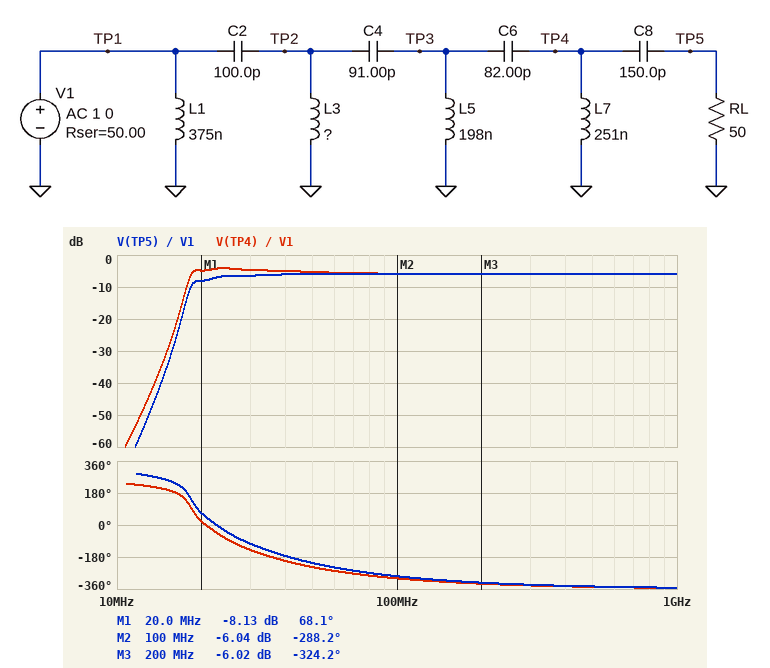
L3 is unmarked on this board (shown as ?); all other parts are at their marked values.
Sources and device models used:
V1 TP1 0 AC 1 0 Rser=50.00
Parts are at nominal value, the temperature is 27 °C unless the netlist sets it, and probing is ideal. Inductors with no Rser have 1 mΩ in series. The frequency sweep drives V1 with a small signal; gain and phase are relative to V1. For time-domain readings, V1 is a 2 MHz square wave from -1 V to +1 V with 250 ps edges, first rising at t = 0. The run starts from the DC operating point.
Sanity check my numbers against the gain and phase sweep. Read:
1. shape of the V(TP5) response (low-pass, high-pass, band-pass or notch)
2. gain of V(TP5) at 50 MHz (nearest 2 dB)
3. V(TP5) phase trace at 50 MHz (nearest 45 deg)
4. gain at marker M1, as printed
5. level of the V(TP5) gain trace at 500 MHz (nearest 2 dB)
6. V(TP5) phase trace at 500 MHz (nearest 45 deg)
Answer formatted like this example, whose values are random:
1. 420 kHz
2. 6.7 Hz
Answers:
1. high-pass
2. -6 dB
3. -225 deg
4. -8.13 dB
5. -6 dB
6. -360 deg
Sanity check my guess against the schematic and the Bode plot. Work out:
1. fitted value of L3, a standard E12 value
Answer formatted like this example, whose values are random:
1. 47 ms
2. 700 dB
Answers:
1. 270 nH
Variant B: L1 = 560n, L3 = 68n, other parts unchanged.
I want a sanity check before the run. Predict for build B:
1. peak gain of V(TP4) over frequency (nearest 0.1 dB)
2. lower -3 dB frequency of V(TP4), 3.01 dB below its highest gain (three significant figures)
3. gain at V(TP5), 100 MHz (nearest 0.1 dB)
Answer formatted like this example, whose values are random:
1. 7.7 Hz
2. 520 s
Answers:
1. -6.0 dB
2. 31.6 MHz
3. -6.8 dB
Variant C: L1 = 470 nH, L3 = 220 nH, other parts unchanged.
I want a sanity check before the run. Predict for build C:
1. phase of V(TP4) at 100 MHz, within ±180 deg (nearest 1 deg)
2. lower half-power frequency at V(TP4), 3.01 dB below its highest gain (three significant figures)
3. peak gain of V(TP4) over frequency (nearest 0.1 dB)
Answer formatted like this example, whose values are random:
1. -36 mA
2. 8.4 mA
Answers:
1. 61 deg
2. 19.2 MHz
3. -3.1 dB
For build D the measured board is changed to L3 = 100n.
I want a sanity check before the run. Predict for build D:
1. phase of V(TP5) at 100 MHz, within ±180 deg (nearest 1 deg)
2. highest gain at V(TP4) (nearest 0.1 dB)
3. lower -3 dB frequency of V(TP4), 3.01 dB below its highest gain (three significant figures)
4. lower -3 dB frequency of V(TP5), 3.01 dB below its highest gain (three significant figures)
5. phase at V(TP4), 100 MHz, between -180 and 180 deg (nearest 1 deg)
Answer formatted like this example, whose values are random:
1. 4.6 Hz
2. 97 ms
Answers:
1. 86 deg
2. -5.6 dB
3. 22.3 MHz
4. 26.2 MHz
5. 74 deg
